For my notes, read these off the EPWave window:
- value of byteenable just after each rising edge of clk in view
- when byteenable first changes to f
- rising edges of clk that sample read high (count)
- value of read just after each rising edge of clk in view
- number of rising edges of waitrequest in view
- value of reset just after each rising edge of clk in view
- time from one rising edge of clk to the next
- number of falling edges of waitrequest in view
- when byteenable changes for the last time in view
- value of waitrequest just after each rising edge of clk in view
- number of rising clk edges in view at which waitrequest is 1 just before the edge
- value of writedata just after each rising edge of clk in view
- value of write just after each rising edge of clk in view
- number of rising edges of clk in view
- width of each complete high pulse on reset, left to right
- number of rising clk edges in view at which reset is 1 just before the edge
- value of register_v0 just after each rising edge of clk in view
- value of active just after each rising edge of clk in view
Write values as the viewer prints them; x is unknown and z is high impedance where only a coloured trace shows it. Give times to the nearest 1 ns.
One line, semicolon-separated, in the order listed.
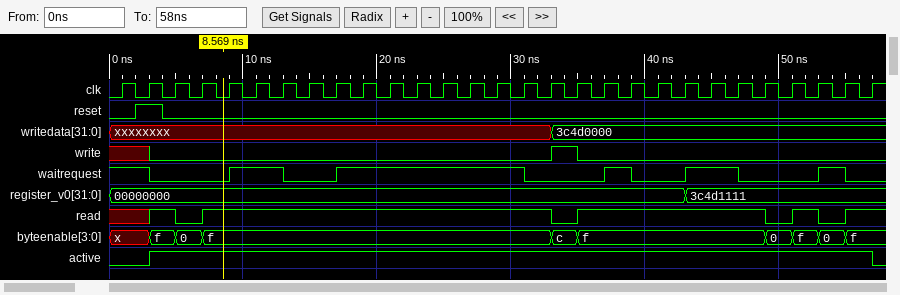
x, f, 0, f, f, f, f, f, f, f, f, f, f, f, f, f, c, f, f, f, f, f, f, f, 0, f, 0, f, f; 3 ns; 23; x 1 0 1 1 1 1 1 1 1 1 1 1 1 1 1 0 1 1 1 1 1 1 1 0 1 0 1 1; 5; 0 1 0 0 0 0 0 0 0 0 0 0 0 0 0 0 0 0 0 0 0 0 0 0 0 0 0 0 0; 2 ns; 6; 55 ns; 1 0 0 0 1 1 0 0 1 1 1 1 1 1 1 0 0 0 1 0 0 1 1 0 0 0 1 0 0; 15; xxxxxxxx, xxxxxxxx, xxxxxxxx, xxxxxxxx, xxxxxxxx, xxxxxxxx, xxxxxxxx, xxxxxxxx, xxxxxxxx, xxxxxxxx, xxxxxxxx, xxxxxxxx, xxxxxxxx, xxxxxxxx, xxxxxxxx, xxxxxxxx, 3c4d0000, 3c4d0000, 3c4d0000, 3c4d0000, 3c4d0000, 3c4d0000, 3c4d0000, 3c4d0000, 3c4d0000, 3c4d0000, 3c4d0000, 3c4d0000, 3c4d0000; x 0 0 0 0 0 0 0 0 0 0 0 0 0 0 0 1 0 0 0 0 0 0 0 0 0 0 0 0; 29; 2 ns; 1; 00000000, 00000000, 00000000, 00000000, 00000000, 00000000, 00000000, 00000000, 00000000, 00000000, 00000000, 00000000, 00000000, 00000000, 00000000, 00000000, 00000000, 00000000, 00000000, 00000000, 00000000, 3c4d1111, 3c4d1111, 3c4d1111, 3c4d1111, 3c4d1111, 3c4d1111, 3c4d1111, 3c4d1111; 0 1 1 1 1 1 1 1 1 1 1 1 1 1 1 1 1 1 1 1 1 1 1 1 1 1 1 1 0
